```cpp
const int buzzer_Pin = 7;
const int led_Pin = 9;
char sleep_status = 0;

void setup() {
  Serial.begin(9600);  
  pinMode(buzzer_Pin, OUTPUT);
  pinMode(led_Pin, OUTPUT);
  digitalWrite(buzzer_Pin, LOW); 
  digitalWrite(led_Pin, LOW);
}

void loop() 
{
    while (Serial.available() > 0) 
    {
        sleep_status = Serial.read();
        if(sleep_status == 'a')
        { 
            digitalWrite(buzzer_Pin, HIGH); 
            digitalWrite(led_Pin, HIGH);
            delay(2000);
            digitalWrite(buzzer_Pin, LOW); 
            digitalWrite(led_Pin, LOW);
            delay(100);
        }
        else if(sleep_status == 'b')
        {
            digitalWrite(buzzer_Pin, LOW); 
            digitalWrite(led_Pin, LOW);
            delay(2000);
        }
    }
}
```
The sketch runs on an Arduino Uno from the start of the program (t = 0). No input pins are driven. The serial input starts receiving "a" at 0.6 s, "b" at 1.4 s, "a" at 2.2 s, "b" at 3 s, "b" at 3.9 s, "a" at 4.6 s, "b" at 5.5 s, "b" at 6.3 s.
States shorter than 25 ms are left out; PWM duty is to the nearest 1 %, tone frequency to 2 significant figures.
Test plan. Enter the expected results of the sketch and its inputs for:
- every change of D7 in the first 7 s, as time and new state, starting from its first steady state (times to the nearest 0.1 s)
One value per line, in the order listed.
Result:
0 s low; 0.6 s high; 2.6 s low; 4.7 s high; 6.7 s low
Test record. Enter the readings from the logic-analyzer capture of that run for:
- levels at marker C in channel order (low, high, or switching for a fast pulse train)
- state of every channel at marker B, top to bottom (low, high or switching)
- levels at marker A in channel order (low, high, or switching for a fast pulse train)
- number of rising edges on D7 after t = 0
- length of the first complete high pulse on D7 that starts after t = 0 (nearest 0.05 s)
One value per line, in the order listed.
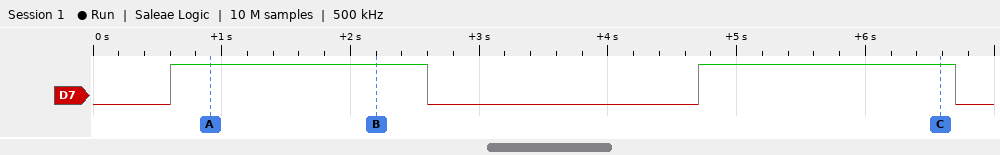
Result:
D7 high
D7 high
D7 high
2
2.00 s
